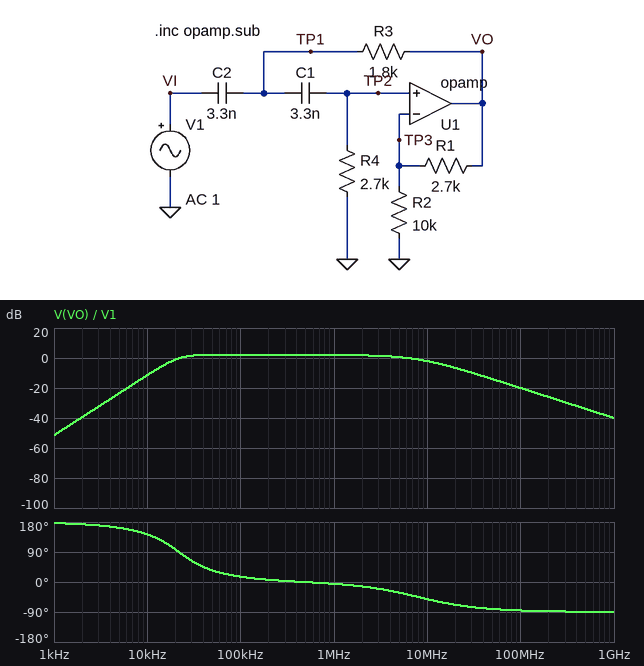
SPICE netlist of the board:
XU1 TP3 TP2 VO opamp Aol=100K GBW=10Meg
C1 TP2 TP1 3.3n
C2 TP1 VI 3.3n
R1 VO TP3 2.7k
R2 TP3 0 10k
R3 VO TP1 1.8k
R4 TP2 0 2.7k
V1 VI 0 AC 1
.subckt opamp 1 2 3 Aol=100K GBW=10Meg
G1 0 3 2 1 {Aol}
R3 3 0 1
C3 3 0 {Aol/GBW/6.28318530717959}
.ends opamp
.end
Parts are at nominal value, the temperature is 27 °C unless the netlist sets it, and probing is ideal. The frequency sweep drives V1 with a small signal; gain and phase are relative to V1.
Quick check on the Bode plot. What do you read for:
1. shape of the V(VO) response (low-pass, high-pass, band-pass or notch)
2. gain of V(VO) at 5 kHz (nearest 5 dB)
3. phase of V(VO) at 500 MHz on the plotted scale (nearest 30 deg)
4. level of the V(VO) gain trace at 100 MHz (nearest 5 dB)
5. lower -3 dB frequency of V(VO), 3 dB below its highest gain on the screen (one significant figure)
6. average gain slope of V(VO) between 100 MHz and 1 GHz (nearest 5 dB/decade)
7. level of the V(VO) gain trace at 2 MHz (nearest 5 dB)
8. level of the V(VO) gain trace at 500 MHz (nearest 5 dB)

band-pass
-25 dB
-90 deg
-20 dB
20 kHz
-20 dB/decade
0 dB
-35 dB
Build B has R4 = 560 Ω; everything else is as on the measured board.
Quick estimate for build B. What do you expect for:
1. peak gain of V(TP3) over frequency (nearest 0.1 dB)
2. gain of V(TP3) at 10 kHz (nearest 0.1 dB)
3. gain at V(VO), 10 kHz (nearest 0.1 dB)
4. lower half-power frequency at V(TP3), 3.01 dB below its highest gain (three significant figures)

-0.2 dB
-28.8 dB
-26.7 dB
145 kHz
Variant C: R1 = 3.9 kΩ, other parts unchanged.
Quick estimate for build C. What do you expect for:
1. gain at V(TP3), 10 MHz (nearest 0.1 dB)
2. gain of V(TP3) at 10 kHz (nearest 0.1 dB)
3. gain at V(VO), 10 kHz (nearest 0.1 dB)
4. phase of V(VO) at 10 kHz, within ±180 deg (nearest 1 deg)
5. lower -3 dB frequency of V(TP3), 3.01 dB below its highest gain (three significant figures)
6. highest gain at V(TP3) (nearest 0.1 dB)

-4.7 dB
-13.2 dB
-10.3 dB
146 deg
19.3 kHz
0.5 dB
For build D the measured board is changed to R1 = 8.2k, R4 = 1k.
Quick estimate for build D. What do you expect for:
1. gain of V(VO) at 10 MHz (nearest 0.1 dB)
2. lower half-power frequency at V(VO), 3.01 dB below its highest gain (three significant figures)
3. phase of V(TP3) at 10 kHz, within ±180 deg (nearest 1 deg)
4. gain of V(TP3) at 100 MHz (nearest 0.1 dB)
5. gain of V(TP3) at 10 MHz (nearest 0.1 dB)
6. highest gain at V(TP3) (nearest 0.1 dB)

-1.2 dB
57.1 kHz
148 deg
-25.2 dB
-6.4 dB
-0.2 dB
